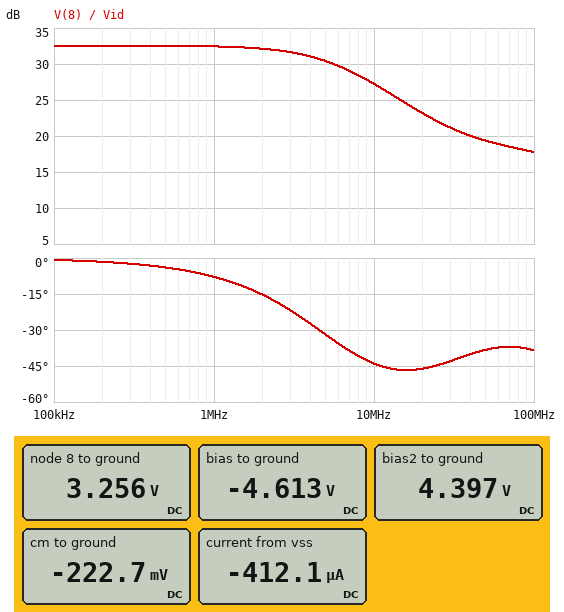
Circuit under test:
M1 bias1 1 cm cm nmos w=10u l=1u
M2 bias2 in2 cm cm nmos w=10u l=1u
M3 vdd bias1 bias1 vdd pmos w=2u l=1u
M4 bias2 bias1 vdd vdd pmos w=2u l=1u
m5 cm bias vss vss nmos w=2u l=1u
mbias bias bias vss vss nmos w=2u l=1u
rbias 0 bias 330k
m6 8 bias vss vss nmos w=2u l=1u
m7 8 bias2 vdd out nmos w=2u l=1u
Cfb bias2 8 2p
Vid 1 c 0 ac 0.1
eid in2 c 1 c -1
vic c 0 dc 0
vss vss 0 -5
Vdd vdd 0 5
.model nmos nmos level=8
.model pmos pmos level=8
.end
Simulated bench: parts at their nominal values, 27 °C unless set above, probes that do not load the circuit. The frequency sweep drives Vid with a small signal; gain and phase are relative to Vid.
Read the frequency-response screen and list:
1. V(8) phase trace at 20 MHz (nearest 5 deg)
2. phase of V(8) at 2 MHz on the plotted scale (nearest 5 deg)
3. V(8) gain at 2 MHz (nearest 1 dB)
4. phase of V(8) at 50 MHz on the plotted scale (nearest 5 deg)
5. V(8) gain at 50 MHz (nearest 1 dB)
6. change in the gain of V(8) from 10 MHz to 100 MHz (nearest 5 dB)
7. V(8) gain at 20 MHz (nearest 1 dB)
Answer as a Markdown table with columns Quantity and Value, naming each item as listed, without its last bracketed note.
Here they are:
| Quantity | Value |
|---|---|
| V(8) phase trace at 20 MHz | -45 deg |
| phase of V(8) at 2 MHz on the plotted scale | -15 deg |
| V(8) gain at 2 MHz | 32 dB |
| phase of V(8) at 50 MHz on the plotted scale | -40 deg |
| V(8) gain at 50 MHz | 19 dB |
| change in the gain of V(8) from 10 MHz to 100 MHz | -10 dB |
| V(8) gain at 20 MHz | 23 dB |
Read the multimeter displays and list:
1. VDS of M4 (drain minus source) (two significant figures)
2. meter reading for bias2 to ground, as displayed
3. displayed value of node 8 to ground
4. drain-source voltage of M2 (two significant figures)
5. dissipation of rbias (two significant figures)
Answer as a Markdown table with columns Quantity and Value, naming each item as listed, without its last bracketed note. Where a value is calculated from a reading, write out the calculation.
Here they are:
| Quantity | Value |
|---|---|
| VDS of M4 (drain minus source) | 4.397 V - 5 V = -600 mV |
| meter reading for bias2 to ground, as displayed | 4.397 V |
| displayed value of node 8 to ground | 3.256 V |
| drain-source voltage of M2 | 4.397 V - (-222.7 mV) = 4.6 V |
| dissipation of rbias | (0 V - (-4.613 V))^2 / 330 kΩ = 64 µW |
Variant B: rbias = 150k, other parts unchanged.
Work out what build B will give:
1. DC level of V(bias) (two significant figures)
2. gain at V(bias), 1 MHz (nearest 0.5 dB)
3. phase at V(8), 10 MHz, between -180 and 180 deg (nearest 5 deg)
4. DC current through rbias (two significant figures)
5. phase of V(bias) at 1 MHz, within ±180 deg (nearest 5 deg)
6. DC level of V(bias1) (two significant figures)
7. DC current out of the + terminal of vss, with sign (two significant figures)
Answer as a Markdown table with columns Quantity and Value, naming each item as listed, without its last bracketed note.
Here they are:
| Quantity | Value |
|---|---|
| DC level of V(bias) | -4.5 V |
| gain at V(bias), 1 MHz | -54.0 dB |
| phase at V(8), 10 MHz, between -180 and 180 deg | -40 deg |
| DC current through rbias | 30 µA |
| phase of V(bias) at 1 MHz, within ±180 deg | 85 deg |
| DC level of V(bias1) | 4.2 V |
| DC current out of the + terminal of vss, with sign | -650 µA |
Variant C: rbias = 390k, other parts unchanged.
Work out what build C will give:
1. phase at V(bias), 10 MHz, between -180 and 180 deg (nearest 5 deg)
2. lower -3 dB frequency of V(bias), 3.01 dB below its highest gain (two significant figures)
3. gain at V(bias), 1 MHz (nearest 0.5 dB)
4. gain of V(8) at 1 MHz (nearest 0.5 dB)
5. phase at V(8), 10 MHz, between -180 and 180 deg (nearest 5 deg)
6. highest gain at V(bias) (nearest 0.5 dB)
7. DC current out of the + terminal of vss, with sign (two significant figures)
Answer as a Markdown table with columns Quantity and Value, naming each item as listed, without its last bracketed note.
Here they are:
| Quantity | Value |
|---|---|
| phase at V(bias), 10 MHz, between -180 and 180 deg | 50 deg |
| lower -3 dB frequency of V(bias), 3.01 dB below its highest gain | 98 MHz |
| gain at V(bias), 1 MHz | -48.0 dB |
| gain of V(8) at 1 MHz | 33.0 dB |
| phase at V(8), 10 MHz, between -180 and 180 deg | -40 deg |
| highest gain at V(bias) | -18.5 dB |
| DC current out of the + terminal of vss, with sign | -370 µA |
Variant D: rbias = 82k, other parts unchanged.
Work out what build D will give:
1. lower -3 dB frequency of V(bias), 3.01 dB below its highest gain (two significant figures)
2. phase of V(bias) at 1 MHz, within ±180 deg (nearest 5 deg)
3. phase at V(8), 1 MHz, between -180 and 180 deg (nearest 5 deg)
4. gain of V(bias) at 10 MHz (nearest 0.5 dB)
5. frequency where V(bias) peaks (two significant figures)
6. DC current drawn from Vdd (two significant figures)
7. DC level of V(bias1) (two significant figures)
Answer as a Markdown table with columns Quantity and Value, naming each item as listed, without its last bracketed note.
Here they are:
| Quantity | Value |
|---|---|
| lower -3 dB frequency of V(bias), 3.01 dB below its highest gain | 310 MHz |
| phase of V(bias) at 1 MHz, within ±180 deg | 85 deg |
| phase at V(8), 1 MHz, between -180 and 180 deg | -5 deg |
| gain of V(bias) at 10 MHz | -41.0 dB |
| frequency where V(bias) peaks | 800 MHz |
| DC current drawn from Vdd | 840 µA |
| DC level of V(bias1) | 4.1 V |
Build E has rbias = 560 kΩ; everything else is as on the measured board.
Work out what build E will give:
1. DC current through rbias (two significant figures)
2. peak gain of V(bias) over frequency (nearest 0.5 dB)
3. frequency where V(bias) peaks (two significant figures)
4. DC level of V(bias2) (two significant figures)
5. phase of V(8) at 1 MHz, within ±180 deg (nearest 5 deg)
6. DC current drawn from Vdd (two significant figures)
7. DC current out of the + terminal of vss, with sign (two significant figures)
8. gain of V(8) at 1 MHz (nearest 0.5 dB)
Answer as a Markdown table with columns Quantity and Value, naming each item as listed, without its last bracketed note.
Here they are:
| Quantity | Value |
|---|---|
| DC current through rbias | 8.3 µA |
| peak gain of V(bias) over frequency | -20.5 dB |
| frequency where V(bias) peaks | 250 MHz |
| DC level of V(bias2) | 4.5 V |
| phase of V(8) at 1 MHz, within ±180 deg | -10 deg |
| DC current drawn from Vdd | 290 µA |
| DC current out of the + terminal of vss, with sign | -300 µA |
| gain of V(8) at 1 MHz | 33.5 dB |
